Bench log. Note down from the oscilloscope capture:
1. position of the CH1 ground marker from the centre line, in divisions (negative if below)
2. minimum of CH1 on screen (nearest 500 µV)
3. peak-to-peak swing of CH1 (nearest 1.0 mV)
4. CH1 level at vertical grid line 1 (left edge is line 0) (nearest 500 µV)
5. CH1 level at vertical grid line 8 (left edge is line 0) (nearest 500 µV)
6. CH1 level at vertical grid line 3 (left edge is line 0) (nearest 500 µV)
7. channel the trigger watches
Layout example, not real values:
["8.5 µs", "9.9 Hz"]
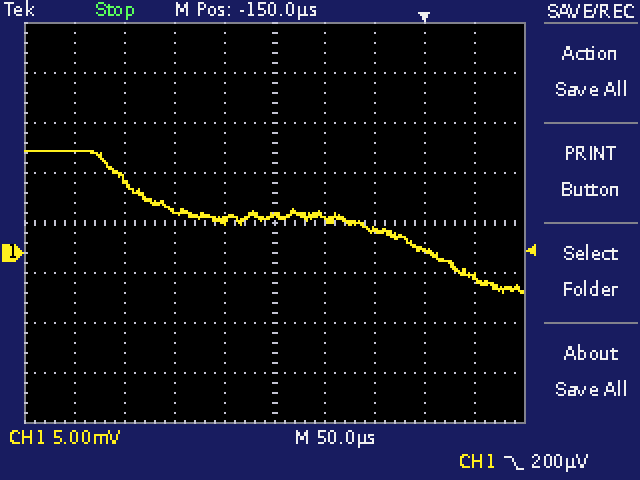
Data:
["-0.6 div", "-4.0 mV", "14.0 mV", "10.0 mV", "500 µV", "4.0 mV", "CH1"]
